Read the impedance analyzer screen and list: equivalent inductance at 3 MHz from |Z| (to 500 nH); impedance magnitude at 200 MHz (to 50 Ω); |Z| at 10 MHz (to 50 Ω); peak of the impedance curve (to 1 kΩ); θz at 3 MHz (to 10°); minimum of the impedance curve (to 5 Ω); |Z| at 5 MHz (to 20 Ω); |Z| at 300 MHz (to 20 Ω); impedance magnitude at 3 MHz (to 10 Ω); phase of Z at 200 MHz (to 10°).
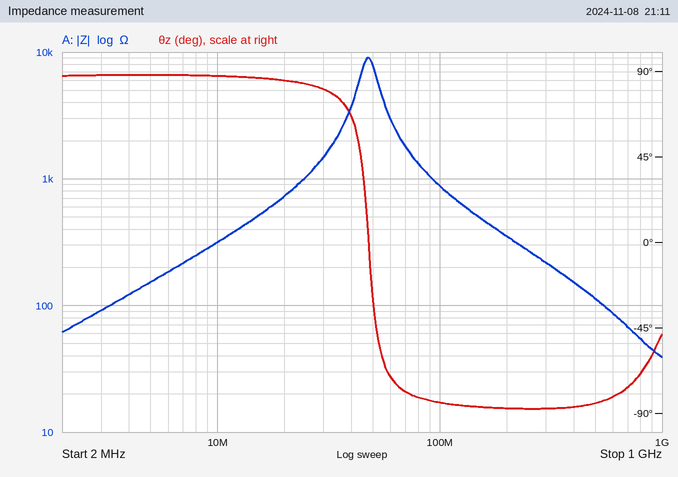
5.0 µH
350 Ω
300 Ω
9 kΩ
90°
40 Ω
160 Ω
220 Ω
90 Ω
-90°
